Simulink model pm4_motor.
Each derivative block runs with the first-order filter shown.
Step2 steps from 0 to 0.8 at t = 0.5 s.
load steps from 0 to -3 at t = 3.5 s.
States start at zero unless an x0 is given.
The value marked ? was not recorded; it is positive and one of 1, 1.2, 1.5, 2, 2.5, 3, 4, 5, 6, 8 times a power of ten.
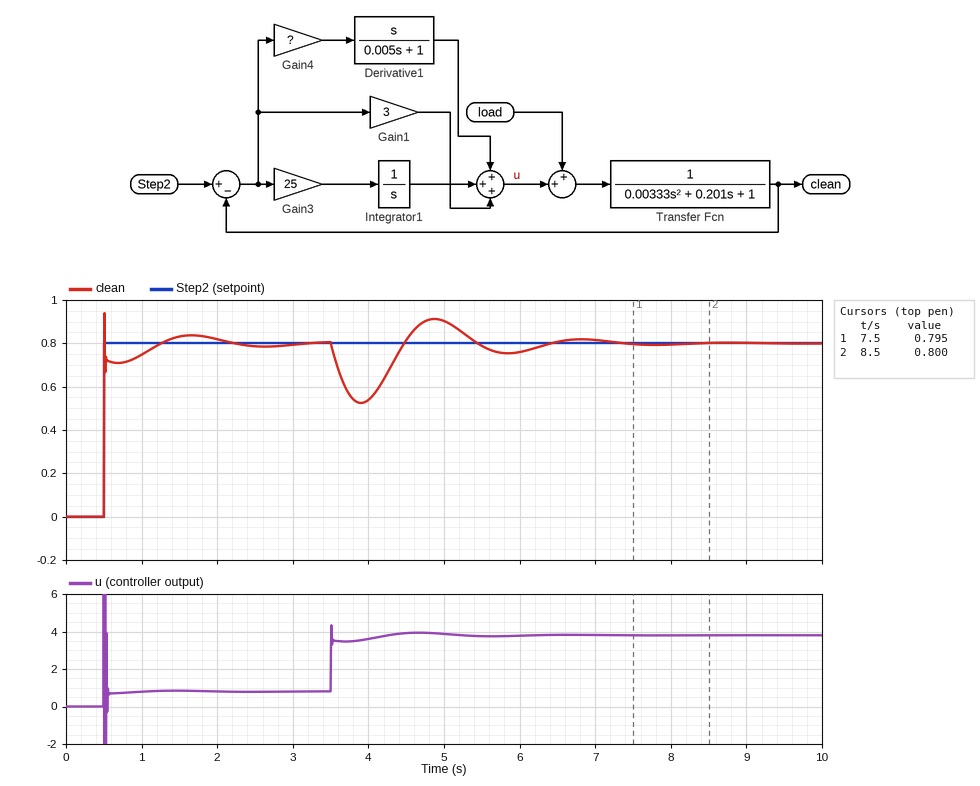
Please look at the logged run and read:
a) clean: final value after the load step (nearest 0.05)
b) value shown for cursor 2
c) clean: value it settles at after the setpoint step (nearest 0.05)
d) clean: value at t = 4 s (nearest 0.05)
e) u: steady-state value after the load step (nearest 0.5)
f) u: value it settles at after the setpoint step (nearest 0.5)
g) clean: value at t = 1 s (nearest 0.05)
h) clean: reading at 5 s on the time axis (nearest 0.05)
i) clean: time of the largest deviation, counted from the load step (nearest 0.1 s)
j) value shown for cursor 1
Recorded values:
0.80
0.800
0.80
0.55
4.0
1.0
0.75
0.90
0.4 s
0.795
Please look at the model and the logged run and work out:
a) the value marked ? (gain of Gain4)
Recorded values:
2
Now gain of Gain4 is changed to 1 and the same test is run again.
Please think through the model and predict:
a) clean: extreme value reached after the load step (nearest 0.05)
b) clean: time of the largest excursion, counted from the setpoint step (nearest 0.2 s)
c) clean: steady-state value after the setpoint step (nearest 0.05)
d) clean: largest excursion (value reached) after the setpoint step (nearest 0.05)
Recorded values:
0.45
0.8 s
0.80
0.85
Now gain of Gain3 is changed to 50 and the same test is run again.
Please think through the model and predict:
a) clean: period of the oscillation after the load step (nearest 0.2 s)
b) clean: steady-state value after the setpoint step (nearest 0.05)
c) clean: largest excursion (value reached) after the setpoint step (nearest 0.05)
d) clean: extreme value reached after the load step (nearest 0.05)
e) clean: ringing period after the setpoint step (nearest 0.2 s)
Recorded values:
1.4 s
0.80
0.95
0.60
0.8 s
